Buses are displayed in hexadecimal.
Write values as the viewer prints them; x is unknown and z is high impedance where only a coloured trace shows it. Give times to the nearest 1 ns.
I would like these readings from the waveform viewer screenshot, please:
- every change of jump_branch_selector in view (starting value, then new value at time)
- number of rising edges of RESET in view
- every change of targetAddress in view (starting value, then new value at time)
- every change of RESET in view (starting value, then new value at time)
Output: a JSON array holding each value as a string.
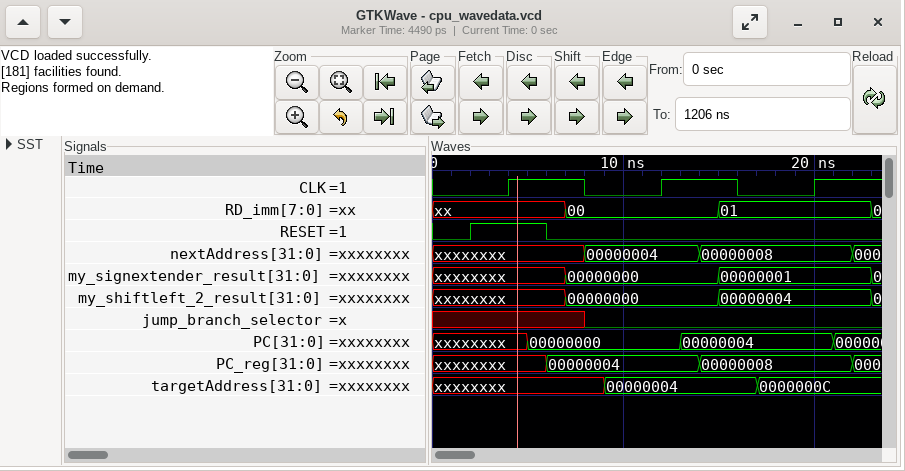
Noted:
["x, 0 at 8 ns", "1", "xxxxxxxx, 00000004 at 9 ns, 0000000C at 17 ns", "0, 1 at 2 ns, 0 at 6 ns"]
